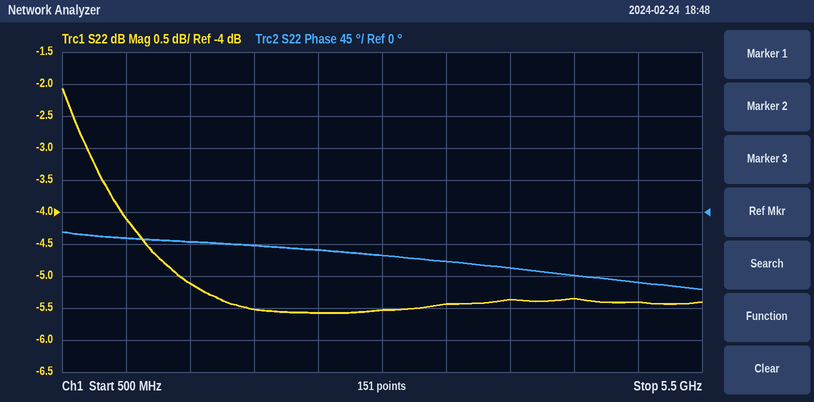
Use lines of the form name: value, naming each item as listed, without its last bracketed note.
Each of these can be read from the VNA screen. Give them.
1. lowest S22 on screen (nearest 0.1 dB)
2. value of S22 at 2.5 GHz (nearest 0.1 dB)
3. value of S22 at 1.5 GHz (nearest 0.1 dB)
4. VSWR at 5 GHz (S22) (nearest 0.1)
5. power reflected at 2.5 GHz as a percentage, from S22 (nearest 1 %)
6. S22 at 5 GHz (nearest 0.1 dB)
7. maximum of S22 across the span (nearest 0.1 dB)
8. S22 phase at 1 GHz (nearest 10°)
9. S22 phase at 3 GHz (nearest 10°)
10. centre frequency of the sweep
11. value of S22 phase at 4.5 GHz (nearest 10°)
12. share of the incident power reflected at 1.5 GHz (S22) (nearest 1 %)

lowest S22 on screen: -5.6 dB
value of S22 at 2.5 GHz: -5.6 dB
value of S22 at 1.5 GHz: -5.1 dB
VSWR at 5 GHz (S22): 3.3
power reflected at 2.5 GHz as a percentage, from S22: 28 %
S22 at 5 GHz: -5.4 dB
maximum of S22 across the span: -2.1 dB
S22 phase at 1 GHz: -40°
S22 phase at 3 GHz: -60°
centre frequency of the sweep: 3 GHz
value of S22 phase at 4.5 GHz: -90°
share of the incident power reflected at 1.5 GHz (S22): 31 %
